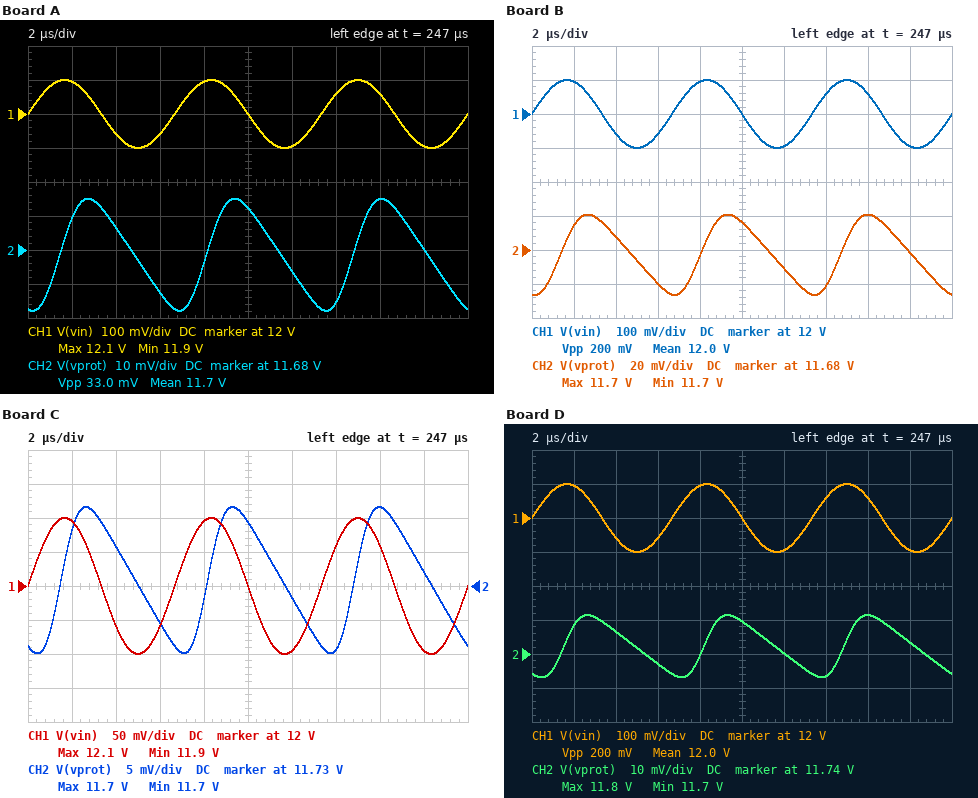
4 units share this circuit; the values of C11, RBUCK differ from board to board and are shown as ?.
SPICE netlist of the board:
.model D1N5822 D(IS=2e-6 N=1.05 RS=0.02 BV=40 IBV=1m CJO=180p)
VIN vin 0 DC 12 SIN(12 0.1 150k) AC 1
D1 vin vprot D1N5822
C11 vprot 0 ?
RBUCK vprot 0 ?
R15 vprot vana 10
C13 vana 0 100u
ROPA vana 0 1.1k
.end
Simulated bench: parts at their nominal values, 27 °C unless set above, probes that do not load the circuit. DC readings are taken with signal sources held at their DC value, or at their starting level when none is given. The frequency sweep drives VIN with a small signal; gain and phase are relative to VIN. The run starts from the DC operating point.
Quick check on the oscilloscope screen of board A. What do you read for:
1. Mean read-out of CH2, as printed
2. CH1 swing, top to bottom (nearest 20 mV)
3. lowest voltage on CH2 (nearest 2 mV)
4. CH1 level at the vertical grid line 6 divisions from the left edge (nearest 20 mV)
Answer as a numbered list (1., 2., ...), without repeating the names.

1. 11.7 V
2. 200 mV
3. 11.662 V
4. 11.90 V
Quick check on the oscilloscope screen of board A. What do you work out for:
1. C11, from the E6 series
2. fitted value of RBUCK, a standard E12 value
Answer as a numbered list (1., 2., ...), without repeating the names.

1. 68 µF
2. 18 Ω
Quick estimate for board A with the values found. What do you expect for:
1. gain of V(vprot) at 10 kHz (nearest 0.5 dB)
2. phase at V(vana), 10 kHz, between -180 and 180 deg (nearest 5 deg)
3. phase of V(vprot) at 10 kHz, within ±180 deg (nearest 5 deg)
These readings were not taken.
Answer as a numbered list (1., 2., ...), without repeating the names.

1. -0.5 dB
2. -105 deg
3. -15 deg
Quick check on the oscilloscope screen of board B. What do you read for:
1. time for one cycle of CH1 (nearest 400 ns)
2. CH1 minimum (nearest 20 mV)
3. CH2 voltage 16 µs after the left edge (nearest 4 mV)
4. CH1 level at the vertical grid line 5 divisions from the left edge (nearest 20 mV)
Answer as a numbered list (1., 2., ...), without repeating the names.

1. 6.8 µs
2. 11.90 V
3. 11.700 V
4. 12.00 V
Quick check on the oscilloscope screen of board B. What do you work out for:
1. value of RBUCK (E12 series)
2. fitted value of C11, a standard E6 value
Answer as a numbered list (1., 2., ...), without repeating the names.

1. 18 Ω
2. 47 µF
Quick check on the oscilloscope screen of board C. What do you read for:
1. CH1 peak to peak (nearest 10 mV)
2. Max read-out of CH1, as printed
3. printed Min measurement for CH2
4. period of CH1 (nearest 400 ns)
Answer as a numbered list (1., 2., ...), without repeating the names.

1. 200 mV
2. 12.1 V
3. 11.7 V
4. 6.8 µs
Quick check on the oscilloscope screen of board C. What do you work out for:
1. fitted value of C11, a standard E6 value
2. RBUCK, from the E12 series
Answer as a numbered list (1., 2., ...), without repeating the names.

1. 33 µF
2. 68 Ω
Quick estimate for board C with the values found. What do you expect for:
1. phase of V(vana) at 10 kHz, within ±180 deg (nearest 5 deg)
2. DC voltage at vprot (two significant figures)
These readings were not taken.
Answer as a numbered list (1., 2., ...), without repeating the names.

1. -110 deg
2. 12 V
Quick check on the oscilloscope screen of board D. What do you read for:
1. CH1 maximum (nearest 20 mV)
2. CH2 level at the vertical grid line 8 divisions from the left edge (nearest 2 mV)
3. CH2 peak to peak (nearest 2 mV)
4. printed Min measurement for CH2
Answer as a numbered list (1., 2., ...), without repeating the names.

1. 12.10 V
2. 11.752 V
3. 18 mV
4. 11.7 V
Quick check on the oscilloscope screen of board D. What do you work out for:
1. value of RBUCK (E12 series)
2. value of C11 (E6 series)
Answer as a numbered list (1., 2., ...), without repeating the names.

1. 82 Ω
2. 33 µF
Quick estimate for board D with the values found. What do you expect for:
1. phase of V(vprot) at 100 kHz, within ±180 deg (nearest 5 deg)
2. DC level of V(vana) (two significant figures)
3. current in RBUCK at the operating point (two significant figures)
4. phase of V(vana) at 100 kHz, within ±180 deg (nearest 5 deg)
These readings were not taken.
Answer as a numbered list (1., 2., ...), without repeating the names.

1. -75 deg
2. 12 V
3. 140 mA
4. -165 deg
